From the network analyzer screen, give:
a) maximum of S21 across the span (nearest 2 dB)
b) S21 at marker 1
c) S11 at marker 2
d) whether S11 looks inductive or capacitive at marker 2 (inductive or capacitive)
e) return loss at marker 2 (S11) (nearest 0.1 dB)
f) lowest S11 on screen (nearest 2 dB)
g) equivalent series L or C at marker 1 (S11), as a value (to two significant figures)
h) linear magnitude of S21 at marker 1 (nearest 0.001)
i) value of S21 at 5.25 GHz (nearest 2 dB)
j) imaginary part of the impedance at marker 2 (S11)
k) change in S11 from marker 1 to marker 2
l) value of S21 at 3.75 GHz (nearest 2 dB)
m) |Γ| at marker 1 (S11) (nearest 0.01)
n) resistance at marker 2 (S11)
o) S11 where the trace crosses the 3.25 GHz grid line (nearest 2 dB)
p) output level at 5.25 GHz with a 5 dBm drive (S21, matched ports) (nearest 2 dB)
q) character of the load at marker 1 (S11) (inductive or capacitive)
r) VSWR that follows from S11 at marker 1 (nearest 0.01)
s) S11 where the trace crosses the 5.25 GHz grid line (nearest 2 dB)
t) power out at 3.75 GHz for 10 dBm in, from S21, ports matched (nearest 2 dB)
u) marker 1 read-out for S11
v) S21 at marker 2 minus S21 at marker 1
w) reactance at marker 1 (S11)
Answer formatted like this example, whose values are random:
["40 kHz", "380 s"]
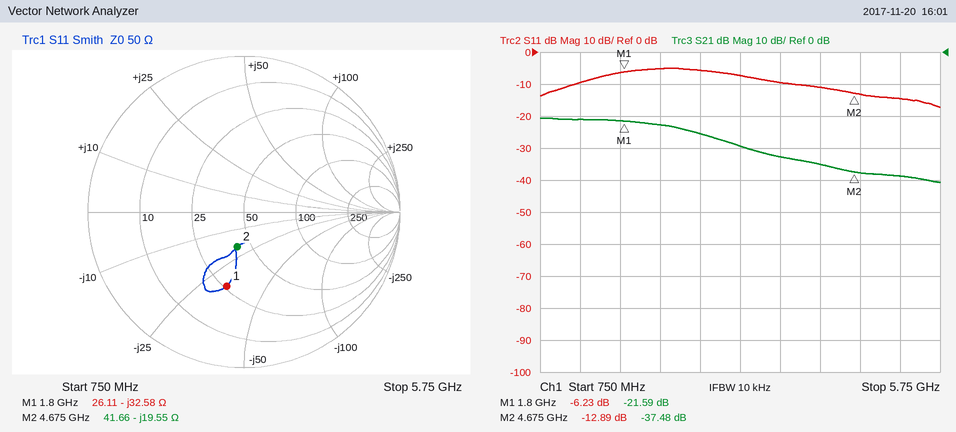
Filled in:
["-20 dB", "-21.59 dB", "-12.89 dB", "capacitive", "12.9 dB", "-18 dB", "2.7 pF", "0.083", "-38 dB", "-19.55 Ω", "-6.66 dB", "-32 dB", "0.49", "41.66 Ω", "-8 dB", "-34 dBm", "capacitive", "2.91", "-14 dB", "-22 dBm", "-6.23 dB", "-15.89 dB", "-32.58 Ω"]
